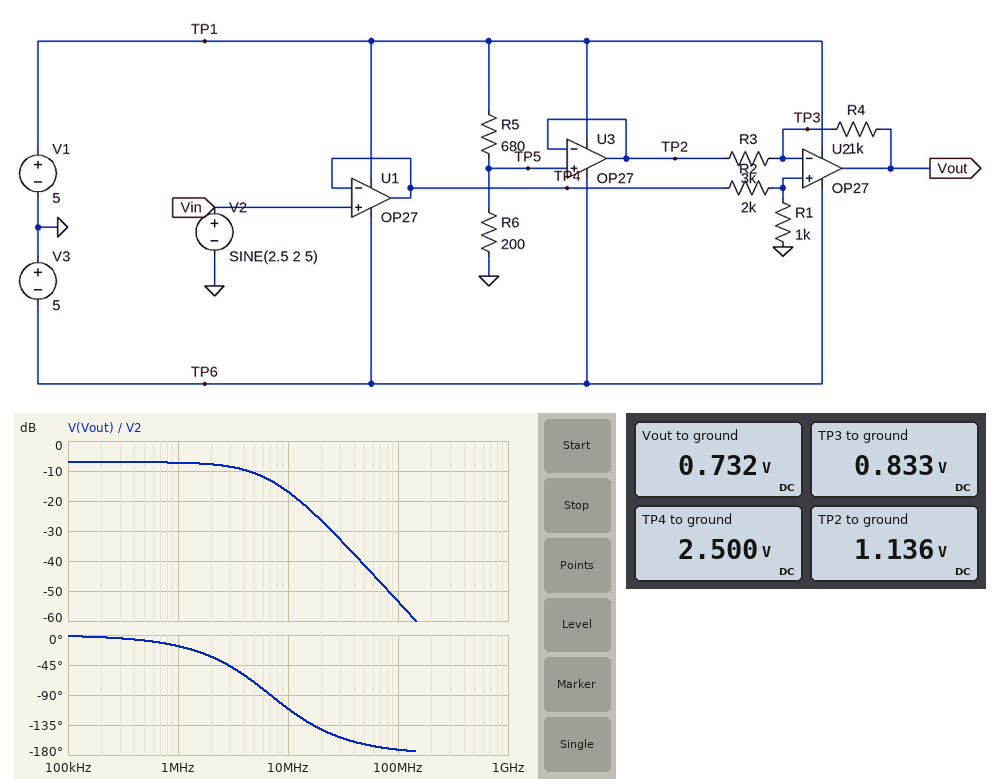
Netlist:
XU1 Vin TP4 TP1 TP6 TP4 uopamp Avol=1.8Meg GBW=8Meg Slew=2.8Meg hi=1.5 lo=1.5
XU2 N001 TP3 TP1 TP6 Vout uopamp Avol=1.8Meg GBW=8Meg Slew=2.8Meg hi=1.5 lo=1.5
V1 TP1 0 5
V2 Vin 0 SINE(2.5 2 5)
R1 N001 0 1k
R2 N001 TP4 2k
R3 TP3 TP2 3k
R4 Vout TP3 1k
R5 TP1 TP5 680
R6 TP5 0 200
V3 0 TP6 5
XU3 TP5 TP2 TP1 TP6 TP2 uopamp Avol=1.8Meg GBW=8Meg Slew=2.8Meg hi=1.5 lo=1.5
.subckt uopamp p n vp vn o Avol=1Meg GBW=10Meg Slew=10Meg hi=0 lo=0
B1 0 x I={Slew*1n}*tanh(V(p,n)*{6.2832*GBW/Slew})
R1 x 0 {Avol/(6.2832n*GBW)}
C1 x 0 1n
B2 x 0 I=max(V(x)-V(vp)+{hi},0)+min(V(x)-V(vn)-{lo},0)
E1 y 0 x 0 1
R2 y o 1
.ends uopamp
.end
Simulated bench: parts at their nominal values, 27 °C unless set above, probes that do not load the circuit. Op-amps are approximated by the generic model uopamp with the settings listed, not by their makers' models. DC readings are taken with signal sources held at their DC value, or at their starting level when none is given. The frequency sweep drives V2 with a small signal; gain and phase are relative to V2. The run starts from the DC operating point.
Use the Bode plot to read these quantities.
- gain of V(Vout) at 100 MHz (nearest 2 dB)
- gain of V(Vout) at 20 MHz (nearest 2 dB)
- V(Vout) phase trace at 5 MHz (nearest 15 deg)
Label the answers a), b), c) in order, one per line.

a) -54 dB
b) -26 dB
c) -75 deg
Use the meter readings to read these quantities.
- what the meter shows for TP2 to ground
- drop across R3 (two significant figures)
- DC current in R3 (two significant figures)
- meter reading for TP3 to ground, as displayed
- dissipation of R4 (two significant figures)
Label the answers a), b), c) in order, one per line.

a) 1.136 V
b) 300 mV
c) 100 µA
d) 0.833 V
e) 10 µW
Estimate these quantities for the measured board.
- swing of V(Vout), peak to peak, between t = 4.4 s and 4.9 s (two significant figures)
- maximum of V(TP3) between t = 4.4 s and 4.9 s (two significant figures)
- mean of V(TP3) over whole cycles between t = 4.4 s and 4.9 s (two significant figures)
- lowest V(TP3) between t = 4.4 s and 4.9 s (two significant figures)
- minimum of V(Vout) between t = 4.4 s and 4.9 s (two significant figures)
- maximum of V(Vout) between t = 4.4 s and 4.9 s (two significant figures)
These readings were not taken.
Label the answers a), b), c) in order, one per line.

a) 1.3 V
b) 1.2 V
c) 760 mV
d) 170 mV
e) -160 mV
f) 1.2 V
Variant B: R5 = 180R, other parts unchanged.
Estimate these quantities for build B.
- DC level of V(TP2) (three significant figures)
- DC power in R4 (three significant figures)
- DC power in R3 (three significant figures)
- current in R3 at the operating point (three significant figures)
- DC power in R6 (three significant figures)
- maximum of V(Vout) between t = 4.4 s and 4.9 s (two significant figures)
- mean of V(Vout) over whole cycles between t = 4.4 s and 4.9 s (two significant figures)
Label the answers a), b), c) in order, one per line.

a) 2.63 V
b) 359 µW
c) 1.08 mW
d) 599 µA
e) 34.6 mW
f) 680 mV
g) 140 mV
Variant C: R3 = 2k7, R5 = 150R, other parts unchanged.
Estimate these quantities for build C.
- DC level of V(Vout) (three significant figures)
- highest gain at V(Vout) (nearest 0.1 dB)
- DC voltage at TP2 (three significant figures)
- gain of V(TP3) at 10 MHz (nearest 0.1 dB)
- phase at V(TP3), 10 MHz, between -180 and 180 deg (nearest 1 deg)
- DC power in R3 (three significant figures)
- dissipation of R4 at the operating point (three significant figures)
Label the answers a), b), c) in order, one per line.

a) 83.8 mV
b) -6.8 dB
c) 2.86 V
d) -19.6 dB
e) -111 deg
f) 1.52 mW
g) 562 µW
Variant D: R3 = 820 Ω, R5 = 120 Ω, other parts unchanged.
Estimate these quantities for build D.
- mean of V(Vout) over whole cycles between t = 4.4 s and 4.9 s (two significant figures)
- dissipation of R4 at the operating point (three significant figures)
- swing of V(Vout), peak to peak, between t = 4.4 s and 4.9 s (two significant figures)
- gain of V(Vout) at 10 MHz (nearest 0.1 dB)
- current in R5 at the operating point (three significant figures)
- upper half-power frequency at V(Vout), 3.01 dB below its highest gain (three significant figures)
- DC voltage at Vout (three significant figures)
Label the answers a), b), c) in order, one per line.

a) -2.1 V
b) 7.81 mW
c) 2.2 V
d) -16.1 dB
e) 15.6 mA
f) 3.10 MHz
g) -1.96 V
